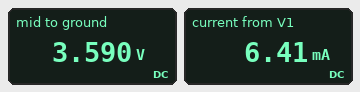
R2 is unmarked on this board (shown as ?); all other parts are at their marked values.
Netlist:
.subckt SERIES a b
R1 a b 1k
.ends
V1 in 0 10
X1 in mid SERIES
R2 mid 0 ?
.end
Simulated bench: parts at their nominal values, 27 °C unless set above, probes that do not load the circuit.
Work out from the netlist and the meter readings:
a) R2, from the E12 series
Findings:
560 Ω
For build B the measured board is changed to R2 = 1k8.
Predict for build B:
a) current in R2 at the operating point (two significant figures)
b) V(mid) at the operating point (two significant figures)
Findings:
3.6 mA
6.4 V
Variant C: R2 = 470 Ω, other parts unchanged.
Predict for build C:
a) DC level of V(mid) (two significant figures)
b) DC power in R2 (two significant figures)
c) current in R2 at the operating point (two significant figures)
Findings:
3.2 V
22 mW
6.8 mA
